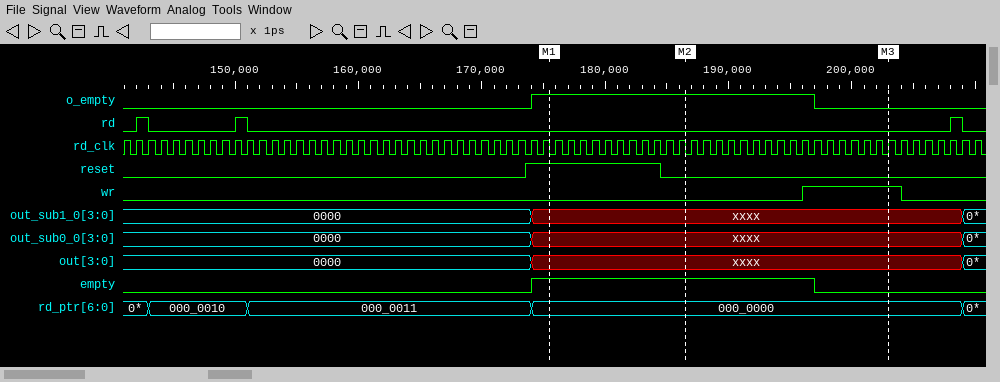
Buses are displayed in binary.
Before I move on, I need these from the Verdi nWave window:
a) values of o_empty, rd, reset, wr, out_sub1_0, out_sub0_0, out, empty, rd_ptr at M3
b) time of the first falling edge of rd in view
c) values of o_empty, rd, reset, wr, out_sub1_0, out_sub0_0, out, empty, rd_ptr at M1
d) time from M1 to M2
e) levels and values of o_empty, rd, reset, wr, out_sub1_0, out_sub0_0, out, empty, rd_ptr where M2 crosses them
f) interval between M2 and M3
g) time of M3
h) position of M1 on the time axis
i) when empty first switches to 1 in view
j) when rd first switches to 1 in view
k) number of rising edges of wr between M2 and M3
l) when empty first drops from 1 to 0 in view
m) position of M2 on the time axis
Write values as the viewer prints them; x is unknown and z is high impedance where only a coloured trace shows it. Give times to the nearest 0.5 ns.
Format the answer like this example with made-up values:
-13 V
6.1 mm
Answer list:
o_empty=0, rd=0, reset=0, wr=1, out_sub1_0=xxxx, out_sub0_0=xxxx, out=xxxx, empty=0, rd_ptr=000_0000
143 ns
o_empty=1, rd=0, reset=1, wr=0, out_sub1_0=xxxx, out_sub0_0=xxxx, out=xxxx, empty=1, rd_ptr=000_0000
11 ns
o_empty=1, rd=0, reset=0, wr=0, out_sub1_0=xxxx, out_sub0_0=xxxx, out=xxxx, empty=1, rd_ptr=000_0000
16.5 ns
203 ns
175.5 ns
174 ns
142 ns
1
197 ns
186.5 ns
